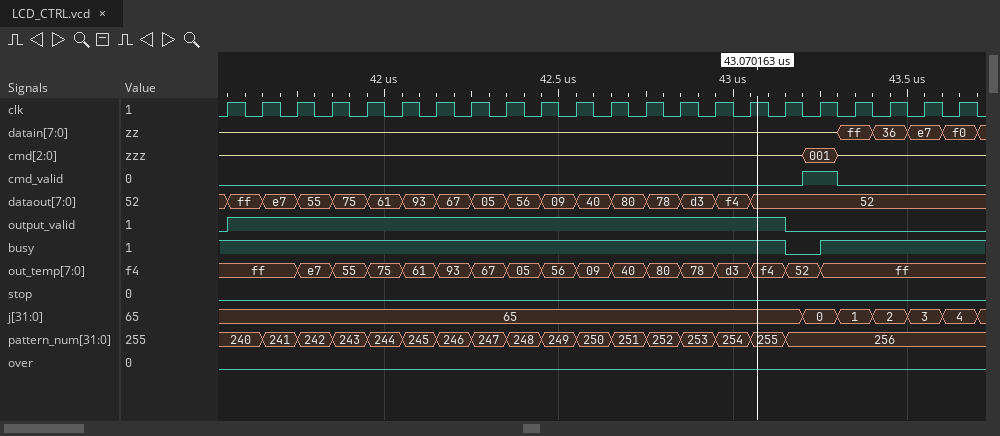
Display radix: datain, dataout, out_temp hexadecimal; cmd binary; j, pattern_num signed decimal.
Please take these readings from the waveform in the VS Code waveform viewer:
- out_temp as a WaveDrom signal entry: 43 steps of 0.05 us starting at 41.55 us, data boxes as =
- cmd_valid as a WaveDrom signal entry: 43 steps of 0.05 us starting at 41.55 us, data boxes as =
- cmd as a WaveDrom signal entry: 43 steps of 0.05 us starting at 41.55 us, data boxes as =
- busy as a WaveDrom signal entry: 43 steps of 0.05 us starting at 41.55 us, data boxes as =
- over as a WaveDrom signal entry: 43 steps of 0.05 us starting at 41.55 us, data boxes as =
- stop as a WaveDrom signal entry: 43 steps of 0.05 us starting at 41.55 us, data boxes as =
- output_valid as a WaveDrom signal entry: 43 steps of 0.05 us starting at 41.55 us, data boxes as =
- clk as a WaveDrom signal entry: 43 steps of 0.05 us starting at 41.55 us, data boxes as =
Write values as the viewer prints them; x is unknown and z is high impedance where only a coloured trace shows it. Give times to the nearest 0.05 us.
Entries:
{name: 'out_temp', wave: '=...=.=.=.=.=.=.=.=.=.=.=.=.=.=.=.=........', data: 'ff e7 55 75 61 93 67 05 56 09 40 80 78 d3 f4 52 ff'}
{name: 'cmd_valid', wave: '0................................1.0.......'}
{name: 'cmd', wave: 'z................................=.z.......', data: '001'}
{name: 'busy', wave: '1...............................0.1........'}
{name: 'over', wave: '0..........................................'}
{name: 'stop', wave: '0..........................................'}
{name: 'output_valid', wave: '1...............................0..........'}
{name: 'clk', wave: '1010101010101010101010101010101010101010101'}
